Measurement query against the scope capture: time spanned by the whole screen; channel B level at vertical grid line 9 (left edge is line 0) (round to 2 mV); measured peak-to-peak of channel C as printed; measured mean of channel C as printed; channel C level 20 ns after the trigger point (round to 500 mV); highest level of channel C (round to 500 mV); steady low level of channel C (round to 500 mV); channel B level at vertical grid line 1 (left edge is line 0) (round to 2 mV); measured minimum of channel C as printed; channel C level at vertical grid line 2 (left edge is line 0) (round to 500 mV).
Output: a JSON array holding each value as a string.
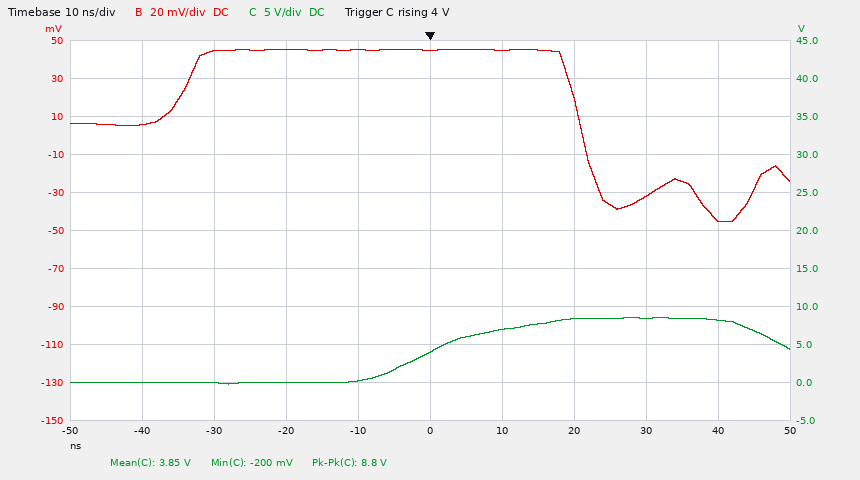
["100 ns", "-44 mV", "8.8 V", "3.85 V", "8.5 V", "8.5 V", "0.0 V", "6 mV", "-200 mV", "0.0 V"]
